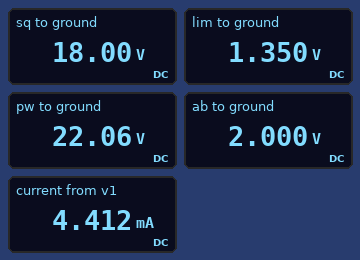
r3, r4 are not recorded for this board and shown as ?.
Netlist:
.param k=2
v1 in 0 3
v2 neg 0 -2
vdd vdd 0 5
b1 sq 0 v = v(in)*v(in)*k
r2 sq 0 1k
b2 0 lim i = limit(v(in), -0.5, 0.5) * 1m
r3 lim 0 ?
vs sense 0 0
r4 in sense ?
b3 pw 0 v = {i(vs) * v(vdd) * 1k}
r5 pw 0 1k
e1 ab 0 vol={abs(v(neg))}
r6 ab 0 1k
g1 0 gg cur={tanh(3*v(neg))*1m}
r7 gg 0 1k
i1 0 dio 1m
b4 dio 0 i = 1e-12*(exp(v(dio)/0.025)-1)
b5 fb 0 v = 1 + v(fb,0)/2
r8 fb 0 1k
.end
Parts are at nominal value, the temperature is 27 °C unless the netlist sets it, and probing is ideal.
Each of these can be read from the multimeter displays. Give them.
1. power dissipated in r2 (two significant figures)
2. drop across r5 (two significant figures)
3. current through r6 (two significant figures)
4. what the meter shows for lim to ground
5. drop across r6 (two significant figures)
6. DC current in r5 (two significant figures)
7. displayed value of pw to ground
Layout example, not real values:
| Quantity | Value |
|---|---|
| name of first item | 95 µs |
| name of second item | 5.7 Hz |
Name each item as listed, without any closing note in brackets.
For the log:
| Quantity | Value |
|---|---|
| power dissipated in r2 | 320 mW |
| drop across r5 | 22 V |
| current through r6 | 2.0 mA |
| what the meter shows for lim to ground | 1.350 V |
| drop across r6 | 2.0 V |
| DC current in r5 | 22 mA |
| displayed value of pw to ground | 22.06 V |
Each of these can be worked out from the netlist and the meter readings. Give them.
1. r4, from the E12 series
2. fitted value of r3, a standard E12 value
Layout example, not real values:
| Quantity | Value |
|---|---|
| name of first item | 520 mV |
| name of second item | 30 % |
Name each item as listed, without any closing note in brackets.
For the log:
| Quantity | Value |
|---|---|
| r4, from the E12 series | 680 Ω |
| fitted value of r3, a standard E12 value | 2.7 kΩ |
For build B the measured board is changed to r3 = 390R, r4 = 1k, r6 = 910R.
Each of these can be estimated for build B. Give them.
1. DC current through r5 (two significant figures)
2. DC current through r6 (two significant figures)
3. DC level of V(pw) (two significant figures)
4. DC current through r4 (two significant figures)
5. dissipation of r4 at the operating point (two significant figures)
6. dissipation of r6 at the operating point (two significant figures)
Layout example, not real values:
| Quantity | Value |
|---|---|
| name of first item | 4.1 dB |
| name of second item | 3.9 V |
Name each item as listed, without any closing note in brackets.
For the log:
| Quantity | Value |
|---|---|
| DC current through r5 | 15 mA |
| DC current through r6 | 2.2 mA |
| DC level of V(pw) | 15 V |
| DC current through r4 | 3.0 mA |
| dissipation of r4 at the operating point | 9.0 mW |
| dissipation of r6 at the operating point | 4.4 mW |
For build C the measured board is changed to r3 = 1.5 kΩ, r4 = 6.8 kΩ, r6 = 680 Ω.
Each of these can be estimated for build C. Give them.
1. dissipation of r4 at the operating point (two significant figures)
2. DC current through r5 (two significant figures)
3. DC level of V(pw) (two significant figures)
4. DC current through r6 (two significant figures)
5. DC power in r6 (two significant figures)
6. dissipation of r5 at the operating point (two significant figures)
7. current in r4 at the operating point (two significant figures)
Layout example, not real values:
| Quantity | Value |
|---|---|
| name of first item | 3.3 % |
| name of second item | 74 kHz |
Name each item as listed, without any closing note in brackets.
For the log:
| Quantity | Value |
|---|---|
| dissipation of r4 at the operating point | 1.3 mW |
| DC current through r5 | 2.2 mA |
| DC level of V(pw) | 2.2 V |
| DC current through r6 | 2.9 mA |
| DC power in r6 | 5.9 mW |
| dissipation of r5 at the operating point | 4.9 mW |
| current in r4 at the operating point | 440 µA |
